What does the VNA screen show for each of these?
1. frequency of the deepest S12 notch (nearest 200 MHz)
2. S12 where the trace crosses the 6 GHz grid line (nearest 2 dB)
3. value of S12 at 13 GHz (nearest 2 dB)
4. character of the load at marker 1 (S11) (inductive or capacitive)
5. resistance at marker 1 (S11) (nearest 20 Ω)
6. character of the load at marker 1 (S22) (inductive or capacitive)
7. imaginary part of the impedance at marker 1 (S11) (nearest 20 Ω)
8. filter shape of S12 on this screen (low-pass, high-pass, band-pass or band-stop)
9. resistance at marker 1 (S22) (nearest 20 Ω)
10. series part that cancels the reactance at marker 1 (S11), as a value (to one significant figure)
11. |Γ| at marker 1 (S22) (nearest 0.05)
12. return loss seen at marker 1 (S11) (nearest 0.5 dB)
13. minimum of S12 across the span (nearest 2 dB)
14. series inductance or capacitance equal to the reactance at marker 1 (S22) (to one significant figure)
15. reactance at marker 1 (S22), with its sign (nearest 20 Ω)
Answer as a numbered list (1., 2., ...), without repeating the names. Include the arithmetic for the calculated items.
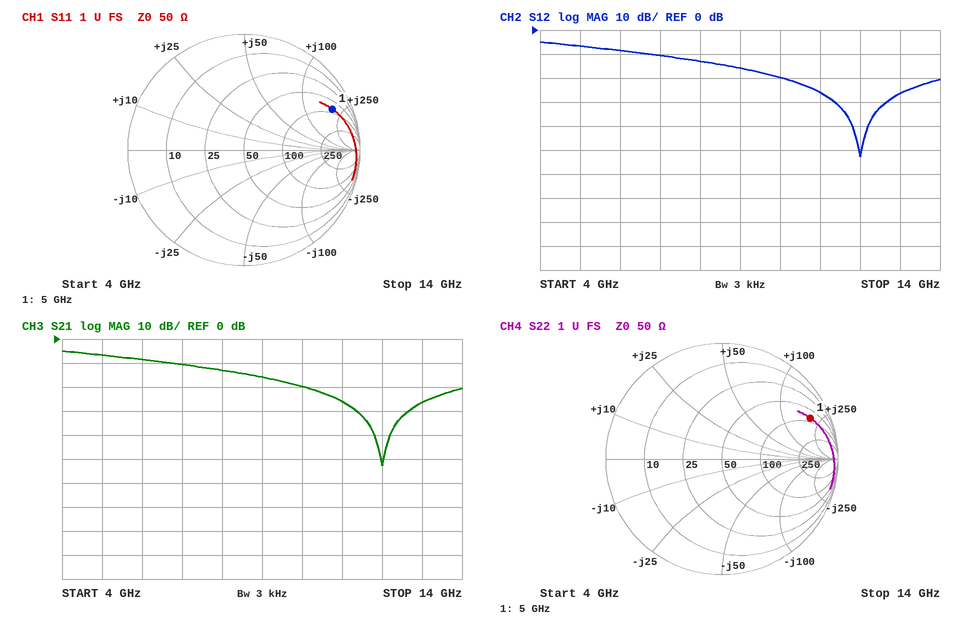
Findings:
1. 12.0 GHz
2. -8 dB
3. -26 dB
4. inductive
5. 80 Ω
6. inductive
7. +200 Ω
8. low-pass
9. 80 Ω
10. C = 1/(2π × 5 GHz × 200 Ω) ≈ 159 fF, so 200 fF to one significant figure
11. 0.85
12. 1.5 dB
13. -52 dB
14. L = 200 Ω/(2π × 5 GHz) ≈ 6 nH
15. +200 Ω
